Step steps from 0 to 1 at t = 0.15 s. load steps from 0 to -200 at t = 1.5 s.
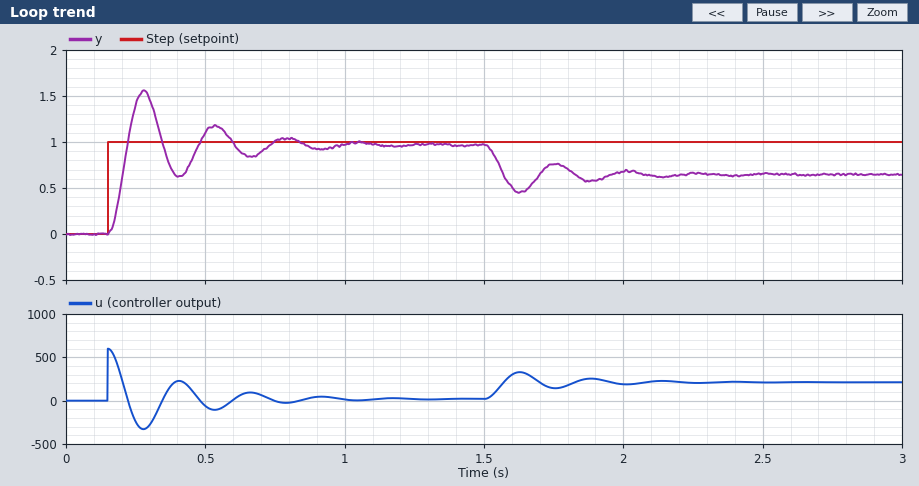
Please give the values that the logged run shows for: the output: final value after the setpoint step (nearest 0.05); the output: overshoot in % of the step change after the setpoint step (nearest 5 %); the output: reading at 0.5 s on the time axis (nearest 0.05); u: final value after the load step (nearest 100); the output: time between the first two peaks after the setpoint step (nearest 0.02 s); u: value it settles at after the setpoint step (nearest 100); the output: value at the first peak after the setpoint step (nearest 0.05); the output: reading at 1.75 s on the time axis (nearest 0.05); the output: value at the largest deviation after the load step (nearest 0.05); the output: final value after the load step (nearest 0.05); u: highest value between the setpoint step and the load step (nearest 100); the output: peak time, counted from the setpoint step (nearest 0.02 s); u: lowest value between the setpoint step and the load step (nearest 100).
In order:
0.95
60 %
1.10
200
0.26 s
0
1.55
0.75
0.45
0.65
600
0.12 s
-300
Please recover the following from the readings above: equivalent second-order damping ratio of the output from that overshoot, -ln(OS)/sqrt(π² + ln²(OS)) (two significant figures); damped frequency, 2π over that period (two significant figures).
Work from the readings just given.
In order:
0.16
24 rad/s
